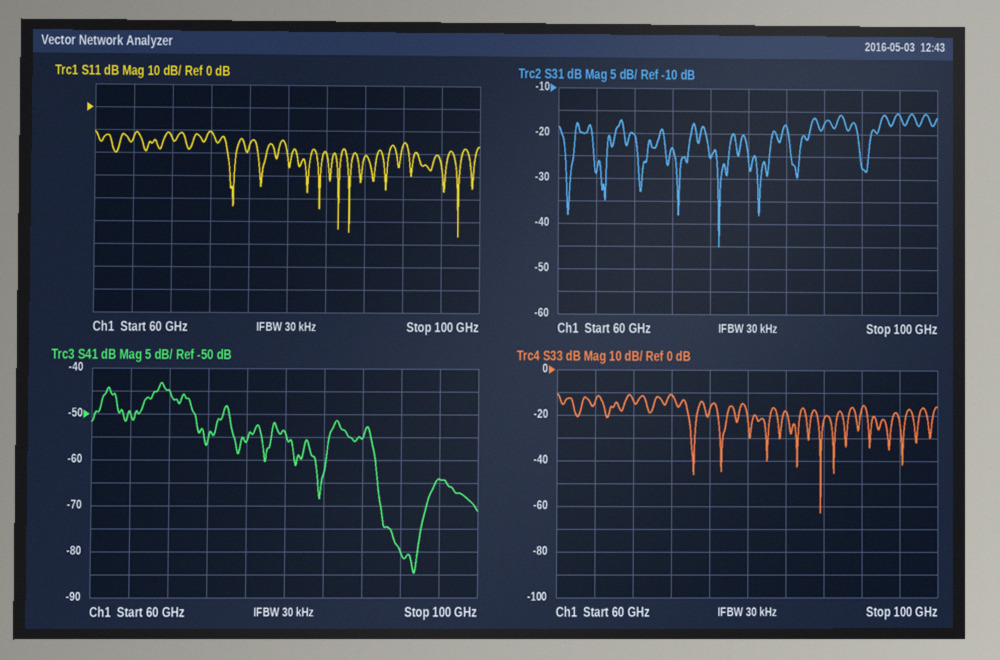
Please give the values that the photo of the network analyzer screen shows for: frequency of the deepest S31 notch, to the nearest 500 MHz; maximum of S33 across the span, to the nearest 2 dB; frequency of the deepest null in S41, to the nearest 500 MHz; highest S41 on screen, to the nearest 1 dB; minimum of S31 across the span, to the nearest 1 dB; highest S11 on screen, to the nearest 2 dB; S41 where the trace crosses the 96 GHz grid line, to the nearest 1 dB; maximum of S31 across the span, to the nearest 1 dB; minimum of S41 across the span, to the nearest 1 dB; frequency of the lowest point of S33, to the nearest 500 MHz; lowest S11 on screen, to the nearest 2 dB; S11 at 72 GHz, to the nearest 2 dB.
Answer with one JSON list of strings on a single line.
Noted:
["77.0 GHz", "-10 dB", "93.5 GHz", "-43 dB", "-45 dB", "-10 dB", "-64 dB", "-15 dB", "-85 dB", "87.5 GHz", "-56 dB", "-10 dB"]
